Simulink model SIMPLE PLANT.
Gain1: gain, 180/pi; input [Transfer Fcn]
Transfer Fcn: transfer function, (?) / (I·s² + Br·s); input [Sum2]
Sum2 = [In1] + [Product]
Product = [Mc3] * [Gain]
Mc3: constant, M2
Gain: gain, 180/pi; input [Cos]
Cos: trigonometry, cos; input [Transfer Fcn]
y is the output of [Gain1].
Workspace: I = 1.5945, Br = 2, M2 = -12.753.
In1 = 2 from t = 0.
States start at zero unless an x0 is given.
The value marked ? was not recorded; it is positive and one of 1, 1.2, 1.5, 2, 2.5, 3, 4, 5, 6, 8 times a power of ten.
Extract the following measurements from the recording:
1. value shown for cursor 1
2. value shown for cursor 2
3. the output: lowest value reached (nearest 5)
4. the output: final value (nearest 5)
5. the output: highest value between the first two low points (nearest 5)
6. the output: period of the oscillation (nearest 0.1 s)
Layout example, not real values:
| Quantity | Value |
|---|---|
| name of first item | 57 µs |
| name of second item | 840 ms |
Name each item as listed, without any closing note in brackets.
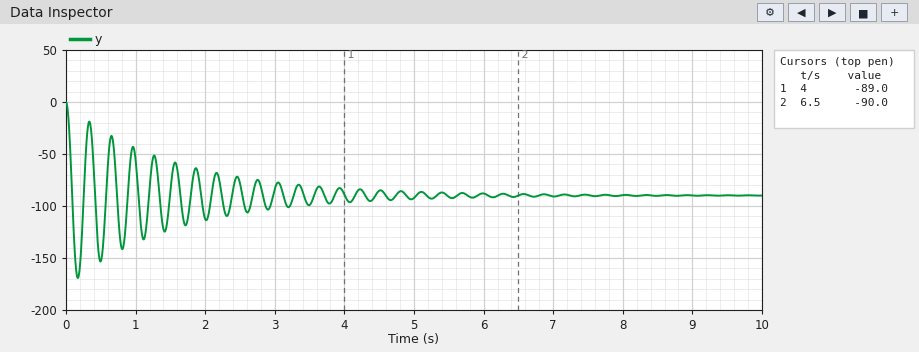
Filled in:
| Quantity | Value |
|---|---|
| value shown for cursor 1 | -89.0 |
| value shown for cursor 2 | -90.0 |
| the output: lowest value reached | -170 |
| the output: final value | -90 |
| the output: highest value between the first two low points | -20 |
| the output: period of the oscillation | 0.3 s |
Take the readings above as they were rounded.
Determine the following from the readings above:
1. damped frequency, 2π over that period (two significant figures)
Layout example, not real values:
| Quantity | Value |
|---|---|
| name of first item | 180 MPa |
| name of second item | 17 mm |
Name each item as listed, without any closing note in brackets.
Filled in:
| Quantity | Value |
|---|---|
| damped frequency, 2π over that period | 21 rad/s |
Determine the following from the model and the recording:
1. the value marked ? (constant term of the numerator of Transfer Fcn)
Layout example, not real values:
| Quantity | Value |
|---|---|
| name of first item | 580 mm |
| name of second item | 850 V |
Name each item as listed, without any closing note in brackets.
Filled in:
| Quantity | Value |
|---|---|
| the value marked ? | 1 |
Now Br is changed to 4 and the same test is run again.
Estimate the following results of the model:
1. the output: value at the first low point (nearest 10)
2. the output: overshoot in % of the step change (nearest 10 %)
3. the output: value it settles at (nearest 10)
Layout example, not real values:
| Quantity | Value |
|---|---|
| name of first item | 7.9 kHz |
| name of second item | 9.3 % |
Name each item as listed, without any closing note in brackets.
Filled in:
| Quantity | Value |
|---|---|
| the output: value at the first low point | -160 |
| the output: overshoot in % of the step change | 80 % |
| the output: value it settles at | -90 |
